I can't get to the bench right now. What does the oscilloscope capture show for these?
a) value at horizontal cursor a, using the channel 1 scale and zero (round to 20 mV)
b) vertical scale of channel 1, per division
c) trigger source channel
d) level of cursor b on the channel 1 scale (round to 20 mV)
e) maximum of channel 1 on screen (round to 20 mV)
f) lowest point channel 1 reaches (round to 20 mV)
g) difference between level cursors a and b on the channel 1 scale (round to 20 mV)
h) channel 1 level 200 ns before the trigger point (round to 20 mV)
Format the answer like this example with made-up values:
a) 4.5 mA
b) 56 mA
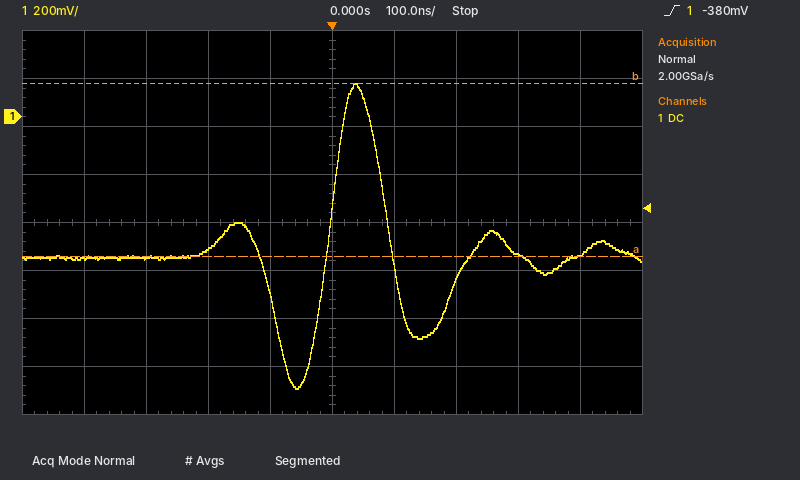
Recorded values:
a) -580 mV
b) 200 mV
c) channel 1
d) 140 mV
e) 140 mV
f) -1.14 V
g) 720 mV
h) -560 mV
